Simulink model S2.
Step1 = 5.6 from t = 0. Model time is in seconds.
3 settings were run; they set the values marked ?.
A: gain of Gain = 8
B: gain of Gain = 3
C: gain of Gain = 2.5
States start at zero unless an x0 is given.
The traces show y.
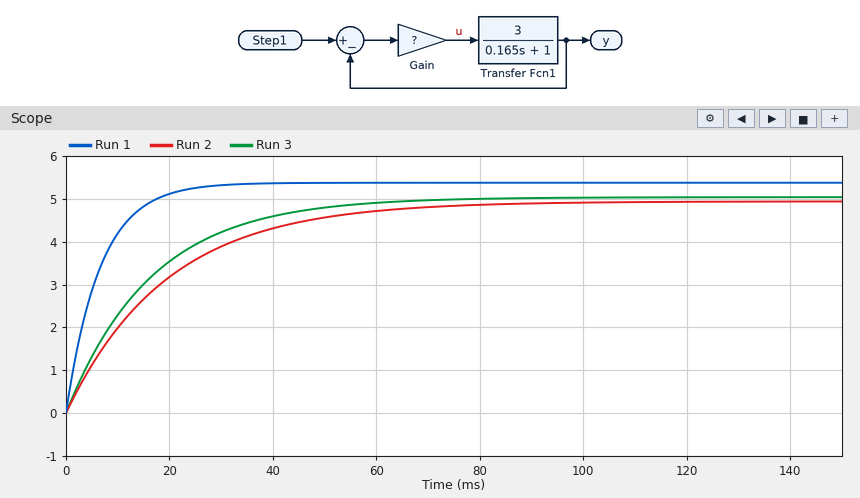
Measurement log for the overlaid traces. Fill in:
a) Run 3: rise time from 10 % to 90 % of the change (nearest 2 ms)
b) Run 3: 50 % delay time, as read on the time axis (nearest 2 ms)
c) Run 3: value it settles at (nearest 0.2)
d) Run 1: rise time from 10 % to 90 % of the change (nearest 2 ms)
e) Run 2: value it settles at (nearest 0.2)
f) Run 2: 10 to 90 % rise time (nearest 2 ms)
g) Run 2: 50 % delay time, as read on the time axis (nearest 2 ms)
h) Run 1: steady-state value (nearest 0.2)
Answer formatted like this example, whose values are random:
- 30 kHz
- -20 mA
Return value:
- 36 ms
- 12 ms
- 5.0
- 14 ms
- 5.0
- 42 ms
- 14 ms
- 5.4
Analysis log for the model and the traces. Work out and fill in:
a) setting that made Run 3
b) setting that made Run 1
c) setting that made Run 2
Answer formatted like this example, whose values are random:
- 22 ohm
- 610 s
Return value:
- B
- A
- C
